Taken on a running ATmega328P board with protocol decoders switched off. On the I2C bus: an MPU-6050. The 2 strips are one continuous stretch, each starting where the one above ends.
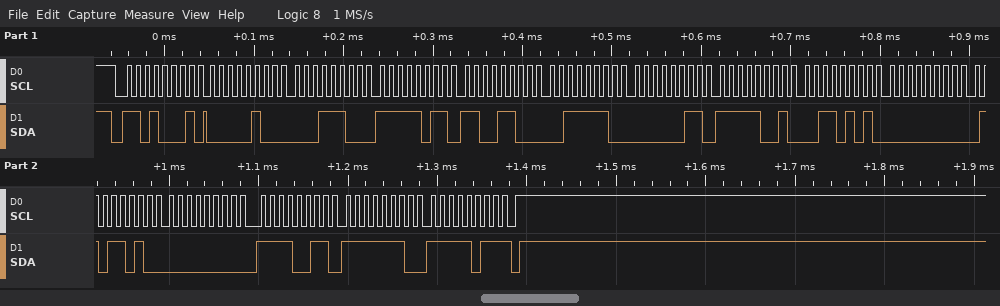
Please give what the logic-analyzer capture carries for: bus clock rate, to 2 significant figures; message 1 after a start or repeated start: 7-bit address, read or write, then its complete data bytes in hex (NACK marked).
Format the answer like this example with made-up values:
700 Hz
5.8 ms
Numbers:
100 kHz
0x68 read: 04 1C FB CC 3E 03 F9 35 00 5A 00 F3 FE FB NACK
